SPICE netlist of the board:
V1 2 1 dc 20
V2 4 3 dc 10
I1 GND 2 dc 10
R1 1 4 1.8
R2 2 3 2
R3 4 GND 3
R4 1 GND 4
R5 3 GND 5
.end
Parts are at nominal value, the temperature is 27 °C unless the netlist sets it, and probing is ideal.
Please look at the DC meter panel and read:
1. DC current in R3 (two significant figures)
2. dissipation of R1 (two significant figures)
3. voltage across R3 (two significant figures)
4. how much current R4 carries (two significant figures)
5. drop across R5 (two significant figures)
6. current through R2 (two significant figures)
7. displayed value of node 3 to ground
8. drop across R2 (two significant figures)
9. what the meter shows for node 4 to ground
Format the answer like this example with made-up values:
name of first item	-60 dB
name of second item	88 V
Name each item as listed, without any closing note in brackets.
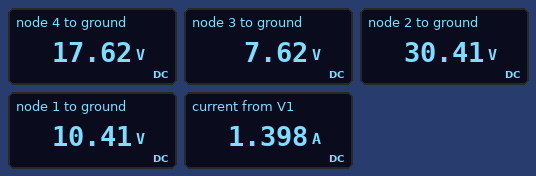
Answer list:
DC current in R3	5.9 A
dissipation of R1	29 W
voltage across R3	18 V
how much current R4 carries	2.6 A
drop across R5	7.6 V
current through R2	11 A
displayed value of node 3 to ground	7.62 V
drop across R2	23 V
what the meter shows for node 4 to ground	17.62 V
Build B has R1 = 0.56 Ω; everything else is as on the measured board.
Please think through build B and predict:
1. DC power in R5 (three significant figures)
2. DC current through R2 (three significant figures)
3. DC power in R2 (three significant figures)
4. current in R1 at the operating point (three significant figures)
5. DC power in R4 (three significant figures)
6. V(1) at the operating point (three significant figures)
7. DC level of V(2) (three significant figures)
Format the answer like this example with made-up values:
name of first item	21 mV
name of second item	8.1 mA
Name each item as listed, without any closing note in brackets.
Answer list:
DC power in R5	8.36 W
DC current through R2	13.2 A
DC power in R2	349 W
current in R1 at the operating point	6.42 A
DC power in R4	41.4 W
V(1) at the operating point	12.9 V
DC level of V(2)	32.9 V
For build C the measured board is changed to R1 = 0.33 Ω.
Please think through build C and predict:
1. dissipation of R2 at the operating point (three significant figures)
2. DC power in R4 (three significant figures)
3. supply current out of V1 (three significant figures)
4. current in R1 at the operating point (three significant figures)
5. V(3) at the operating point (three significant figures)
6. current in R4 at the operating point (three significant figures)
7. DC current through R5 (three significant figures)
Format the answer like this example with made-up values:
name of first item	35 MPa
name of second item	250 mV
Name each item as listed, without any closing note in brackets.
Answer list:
dissipation of R2 at the operating point	381 W
DC power in R4	46.9 W
supply current out of V1	3.81 A
current in R1 at the operating point	7.23 A
V(3) at the operating point	6.08 V
current in R4 at the operating point	3.42 A
DC current through R5	1.22 A
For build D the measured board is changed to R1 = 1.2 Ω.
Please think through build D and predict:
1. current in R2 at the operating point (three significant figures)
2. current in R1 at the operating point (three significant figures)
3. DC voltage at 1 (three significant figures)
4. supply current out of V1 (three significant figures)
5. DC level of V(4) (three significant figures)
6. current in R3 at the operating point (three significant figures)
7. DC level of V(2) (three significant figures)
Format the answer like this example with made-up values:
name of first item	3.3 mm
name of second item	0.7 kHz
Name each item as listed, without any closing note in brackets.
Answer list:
current in R2 at the operating point	12.1 A
current in R1 at the operating point	4.89 A
DC voltage at 1	11.3 V
supply current out of V1	2.06 A
DC level of V(4)	17.2 V
current in R3 at the operating point	5.73 A
DC level of V(2)	31.3 V
